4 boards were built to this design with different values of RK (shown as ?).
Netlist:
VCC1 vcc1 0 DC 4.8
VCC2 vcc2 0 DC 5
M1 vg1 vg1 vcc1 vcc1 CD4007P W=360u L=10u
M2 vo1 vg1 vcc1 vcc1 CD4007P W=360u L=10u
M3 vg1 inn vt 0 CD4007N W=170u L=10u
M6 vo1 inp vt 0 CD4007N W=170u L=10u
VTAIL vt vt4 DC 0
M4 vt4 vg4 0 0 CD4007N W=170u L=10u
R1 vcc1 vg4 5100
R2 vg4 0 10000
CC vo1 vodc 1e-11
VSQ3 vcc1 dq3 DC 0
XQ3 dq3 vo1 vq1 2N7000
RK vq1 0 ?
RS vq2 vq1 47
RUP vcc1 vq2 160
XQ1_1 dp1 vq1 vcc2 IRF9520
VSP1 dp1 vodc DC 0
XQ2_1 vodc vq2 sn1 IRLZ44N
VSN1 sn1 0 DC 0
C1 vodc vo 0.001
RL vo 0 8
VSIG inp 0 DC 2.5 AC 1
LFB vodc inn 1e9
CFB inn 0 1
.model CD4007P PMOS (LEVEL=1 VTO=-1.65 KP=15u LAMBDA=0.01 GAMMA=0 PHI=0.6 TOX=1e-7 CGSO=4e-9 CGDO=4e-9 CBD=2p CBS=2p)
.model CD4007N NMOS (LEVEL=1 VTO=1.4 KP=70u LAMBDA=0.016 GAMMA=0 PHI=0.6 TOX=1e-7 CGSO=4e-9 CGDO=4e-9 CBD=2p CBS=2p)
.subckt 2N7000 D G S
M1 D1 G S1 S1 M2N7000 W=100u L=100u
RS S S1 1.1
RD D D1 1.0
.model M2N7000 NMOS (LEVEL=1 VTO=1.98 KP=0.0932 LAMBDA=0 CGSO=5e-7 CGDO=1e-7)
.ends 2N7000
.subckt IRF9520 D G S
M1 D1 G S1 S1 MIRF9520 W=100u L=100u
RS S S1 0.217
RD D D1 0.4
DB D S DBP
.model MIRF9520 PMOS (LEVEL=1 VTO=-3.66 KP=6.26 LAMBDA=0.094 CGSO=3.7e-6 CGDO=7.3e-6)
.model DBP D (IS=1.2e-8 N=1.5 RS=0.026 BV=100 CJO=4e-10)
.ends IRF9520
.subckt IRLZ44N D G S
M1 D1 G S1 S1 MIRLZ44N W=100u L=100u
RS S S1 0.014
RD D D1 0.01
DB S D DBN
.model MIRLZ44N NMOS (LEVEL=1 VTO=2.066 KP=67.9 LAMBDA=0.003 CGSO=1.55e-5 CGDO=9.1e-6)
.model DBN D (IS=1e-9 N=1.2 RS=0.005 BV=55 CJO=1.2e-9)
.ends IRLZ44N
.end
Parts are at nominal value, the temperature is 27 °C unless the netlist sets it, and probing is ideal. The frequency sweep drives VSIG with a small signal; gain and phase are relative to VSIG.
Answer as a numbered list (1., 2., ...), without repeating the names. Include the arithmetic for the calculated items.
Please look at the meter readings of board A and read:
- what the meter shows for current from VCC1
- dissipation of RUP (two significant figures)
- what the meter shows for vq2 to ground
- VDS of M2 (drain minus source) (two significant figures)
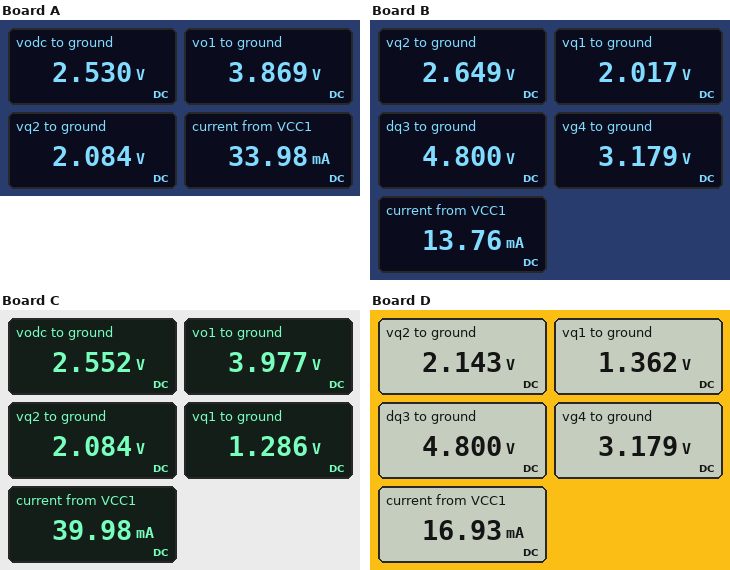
1. 33.98 mA
2. (4.8 V - 2.084 V)^2 / 160 Ω = 46 mW
3. 2.084 V
4. 3.869 V - 4.8 V = -930 mV
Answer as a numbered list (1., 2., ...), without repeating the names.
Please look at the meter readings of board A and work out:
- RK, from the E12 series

1. 39 Ω
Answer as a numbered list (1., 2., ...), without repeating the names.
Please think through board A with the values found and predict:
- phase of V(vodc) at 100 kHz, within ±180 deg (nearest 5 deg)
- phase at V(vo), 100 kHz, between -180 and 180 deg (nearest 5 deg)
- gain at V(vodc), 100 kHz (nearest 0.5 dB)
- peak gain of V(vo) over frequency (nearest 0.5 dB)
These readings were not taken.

1. -45 deg
2. -45 deg
3. 31.0 dB
4. 33.5 dB
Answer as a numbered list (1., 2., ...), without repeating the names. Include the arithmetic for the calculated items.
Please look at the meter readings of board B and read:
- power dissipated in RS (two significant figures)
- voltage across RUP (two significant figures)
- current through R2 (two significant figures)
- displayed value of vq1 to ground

1. (2.649 V - 2.017 V)^2 / 47 Ω = 8.5 mW
2. 4.8 V - 2.649 V = 2.2 V
3. (3.179 V) / 10 kΩ = 320 µA
4. 2.017 V
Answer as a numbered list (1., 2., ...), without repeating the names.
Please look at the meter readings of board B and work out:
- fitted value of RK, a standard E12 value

1. 150 Ω
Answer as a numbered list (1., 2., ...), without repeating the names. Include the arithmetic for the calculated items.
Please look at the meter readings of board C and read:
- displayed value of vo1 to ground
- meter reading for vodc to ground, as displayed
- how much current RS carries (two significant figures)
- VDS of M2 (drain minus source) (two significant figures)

1. 3.977 V
2. 2.552 V
3. (2.084 V - 1.286 V) / 47 Ω = 17 mA
4. 3.977 V - 4.8 V = -820 mV
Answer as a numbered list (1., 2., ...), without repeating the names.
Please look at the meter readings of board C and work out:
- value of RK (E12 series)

1. 33 Ω
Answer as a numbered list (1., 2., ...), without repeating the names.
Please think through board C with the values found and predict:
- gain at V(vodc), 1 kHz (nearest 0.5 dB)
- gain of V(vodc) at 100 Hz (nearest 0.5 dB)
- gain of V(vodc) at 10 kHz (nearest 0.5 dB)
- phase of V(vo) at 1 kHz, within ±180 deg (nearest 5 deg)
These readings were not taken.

1. 29.0 dB
2. 29.5 dB
3. 29.0 dB
4. 0 deg
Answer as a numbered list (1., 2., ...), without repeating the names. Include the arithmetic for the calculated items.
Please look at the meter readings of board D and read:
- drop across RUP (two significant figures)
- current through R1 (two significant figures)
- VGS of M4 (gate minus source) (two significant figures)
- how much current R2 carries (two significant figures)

1. 4.8 V - 2.143 V = 2.7 V
2. (4.8 V - 3.179 V) / 5.1 kΩ = 320 µA
3. 3.179 V = 3.2 V
4. (3.179 V) / 10 kΩ = 320 µA
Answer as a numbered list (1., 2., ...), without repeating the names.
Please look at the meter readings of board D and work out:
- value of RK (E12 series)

1. 82 Ω
